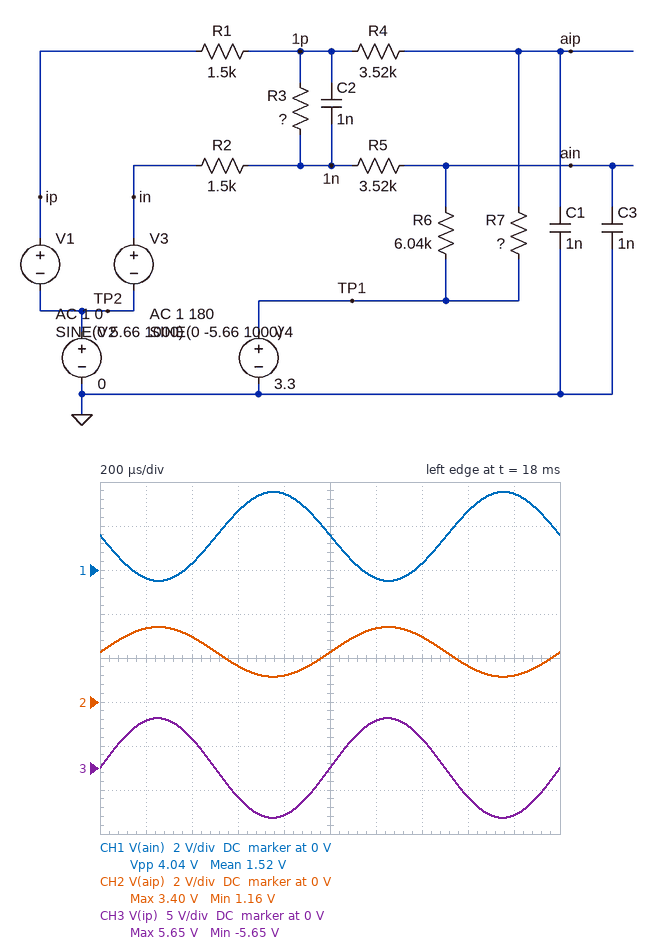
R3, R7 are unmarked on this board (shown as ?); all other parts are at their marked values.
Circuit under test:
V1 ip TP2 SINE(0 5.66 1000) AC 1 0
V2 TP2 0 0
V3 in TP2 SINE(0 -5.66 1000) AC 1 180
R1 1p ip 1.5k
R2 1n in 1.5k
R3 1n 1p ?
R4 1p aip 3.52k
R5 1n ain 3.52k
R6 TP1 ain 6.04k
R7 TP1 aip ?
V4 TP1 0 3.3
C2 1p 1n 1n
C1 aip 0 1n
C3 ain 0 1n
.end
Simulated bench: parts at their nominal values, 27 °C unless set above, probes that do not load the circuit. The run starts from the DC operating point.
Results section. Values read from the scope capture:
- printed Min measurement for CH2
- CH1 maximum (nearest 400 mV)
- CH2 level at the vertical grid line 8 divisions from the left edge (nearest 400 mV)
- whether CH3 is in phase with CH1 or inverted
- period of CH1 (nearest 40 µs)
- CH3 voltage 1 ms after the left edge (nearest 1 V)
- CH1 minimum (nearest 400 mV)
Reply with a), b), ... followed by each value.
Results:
a) 1.16 V
b) 3.6 V
c) 1.6 V
d) inverted
e) 1.00 ms
f) 0 V
g) -400 mV
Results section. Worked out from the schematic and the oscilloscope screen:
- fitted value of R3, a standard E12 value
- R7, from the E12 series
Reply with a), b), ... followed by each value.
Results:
a) 4.7 kΩ
b) 2.2 kΩ
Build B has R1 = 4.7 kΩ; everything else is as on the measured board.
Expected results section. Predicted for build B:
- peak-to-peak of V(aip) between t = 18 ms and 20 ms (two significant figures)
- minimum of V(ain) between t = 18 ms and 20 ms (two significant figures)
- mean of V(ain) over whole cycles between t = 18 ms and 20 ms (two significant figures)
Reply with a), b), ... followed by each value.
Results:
a) 540 mV
b) -730 mV
c) 1.6 V
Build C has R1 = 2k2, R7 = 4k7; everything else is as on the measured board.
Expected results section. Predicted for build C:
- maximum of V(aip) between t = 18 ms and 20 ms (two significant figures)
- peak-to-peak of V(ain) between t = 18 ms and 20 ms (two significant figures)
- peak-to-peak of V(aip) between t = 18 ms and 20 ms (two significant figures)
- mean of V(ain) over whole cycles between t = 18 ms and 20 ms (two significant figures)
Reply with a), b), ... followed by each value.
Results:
a) 3.1 V
b) 4.2 V
c) 2.7 V
d) 1.5 V
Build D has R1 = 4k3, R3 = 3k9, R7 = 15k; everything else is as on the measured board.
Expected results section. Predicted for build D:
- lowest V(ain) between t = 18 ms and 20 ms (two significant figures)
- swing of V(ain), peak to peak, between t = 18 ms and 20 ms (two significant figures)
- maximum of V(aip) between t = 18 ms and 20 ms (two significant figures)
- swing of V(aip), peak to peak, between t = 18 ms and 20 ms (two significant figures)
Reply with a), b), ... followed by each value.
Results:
a) -680 mV
b) 4.4 V
c) 1.7 V
d) 1.3 V
